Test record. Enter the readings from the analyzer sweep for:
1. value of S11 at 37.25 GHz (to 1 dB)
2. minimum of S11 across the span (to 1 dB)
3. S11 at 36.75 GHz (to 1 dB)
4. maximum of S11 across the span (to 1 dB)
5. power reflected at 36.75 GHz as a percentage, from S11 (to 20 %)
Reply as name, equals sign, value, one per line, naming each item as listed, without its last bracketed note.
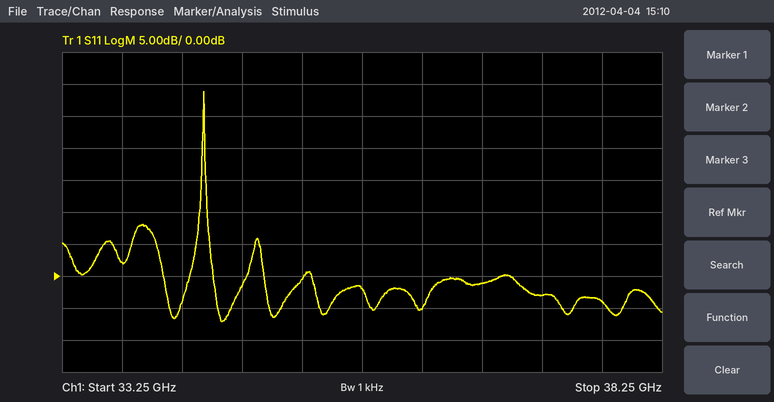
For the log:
value of S11 at 37.25 GHz = -3 dB
minimum of S11 across the span = -7 dB
S11 at 36.75 GHz = -1 dB
maximum of S11 across the span = 29 dB
power reflected at 36.75 GHz as a percentage, from S11 = 80 %
